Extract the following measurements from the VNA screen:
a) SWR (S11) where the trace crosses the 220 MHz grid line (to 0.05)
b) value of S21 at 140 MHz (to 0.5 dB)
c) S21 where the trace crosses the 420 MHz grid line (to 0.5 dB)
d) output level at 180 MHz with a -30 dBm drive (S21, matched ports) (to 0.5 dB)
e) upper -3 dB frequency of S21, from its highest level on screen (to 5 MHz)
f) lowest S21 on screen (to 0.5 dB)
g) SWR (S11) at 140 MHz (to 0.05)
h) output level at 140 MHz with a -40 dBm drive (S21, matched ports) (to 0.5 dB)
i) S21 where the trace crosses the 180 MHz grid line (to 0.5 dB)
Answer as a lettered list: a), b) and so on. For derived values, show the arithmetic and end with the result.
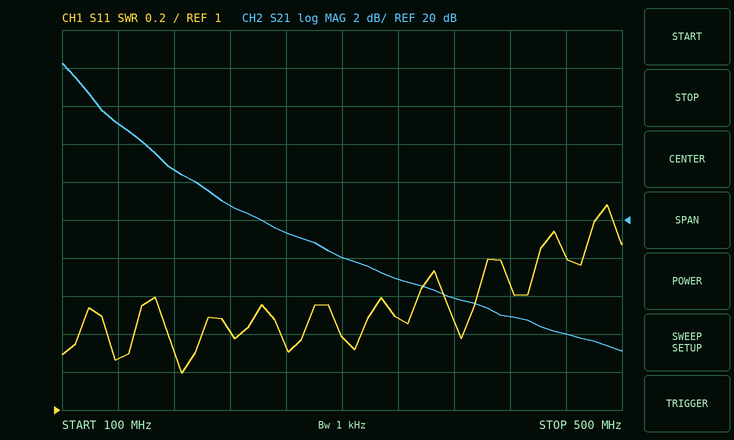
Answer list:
a) 1.40
b) 25.0 dB
c) 15.0 dB
d) -30 dBm + (22.5 dB) = -7.5 dBm
e) 135 MHz
f) 13.0 dB
g) 1.25
h) -40 dBm + (25.0 dB) = -15.0 dBm
i) 22.5 dB
